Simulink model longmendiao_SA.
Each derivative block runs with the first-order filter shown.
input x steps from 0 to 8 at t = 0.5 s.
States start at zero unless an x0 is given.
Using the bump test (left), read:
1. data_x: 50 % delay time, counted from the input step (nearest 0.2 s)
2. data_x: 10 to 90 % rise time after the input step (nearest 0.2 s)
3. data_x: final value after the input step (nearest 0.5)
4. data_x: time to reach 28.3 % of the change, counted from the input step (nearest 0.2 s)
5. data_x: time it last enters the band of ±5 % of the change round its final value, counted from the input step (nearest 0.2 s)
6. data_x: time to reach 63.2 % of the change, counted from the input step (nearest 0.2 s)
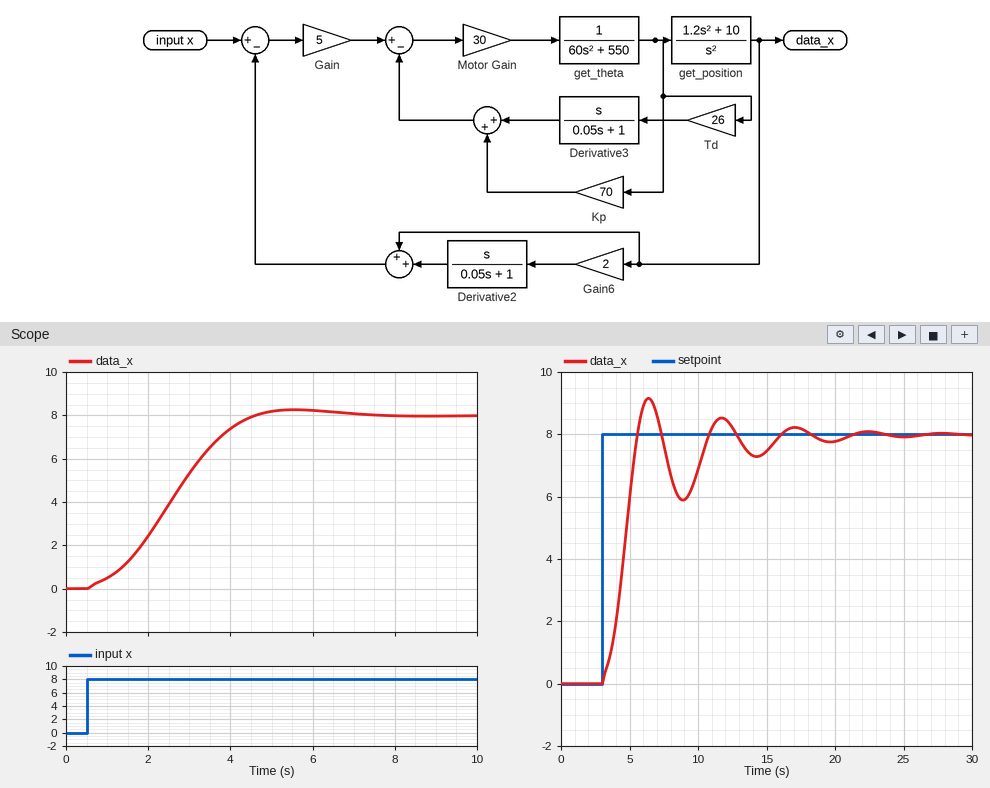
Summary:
2.0 s
2.6 s
8.0
1.4 s
3.6 s
2.4 s
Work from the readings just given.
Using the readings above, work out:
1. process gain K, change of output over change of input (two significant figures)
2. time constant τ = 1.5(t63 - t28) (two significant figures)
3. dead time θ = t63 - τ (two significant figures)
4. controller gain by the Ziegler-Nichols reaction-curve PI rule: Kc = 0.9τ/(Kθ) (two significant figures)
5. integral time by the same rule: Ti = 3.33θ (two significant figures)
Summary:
1.0
1.5 s
0.90 s
1.5
3.0 s
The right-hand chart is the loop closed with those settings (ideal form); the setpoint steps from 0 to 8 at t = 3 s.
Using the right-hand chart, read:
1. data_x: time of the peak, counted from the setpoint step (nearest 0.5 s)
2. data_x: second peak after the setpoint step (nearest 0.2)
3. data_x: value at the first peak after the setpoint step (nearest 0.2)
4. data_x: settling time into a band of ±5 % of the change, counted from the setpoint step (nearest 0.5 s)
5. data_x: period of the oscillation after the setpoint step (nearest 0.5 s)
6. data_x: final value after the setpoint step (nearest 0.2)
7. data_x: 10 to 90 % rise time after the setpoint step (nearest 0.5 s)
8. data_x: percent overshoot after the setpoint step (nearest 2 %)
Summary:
3.5 s
8.6
9.2
12.5 s
5.5 s
8.0
2.0 s
14 %
